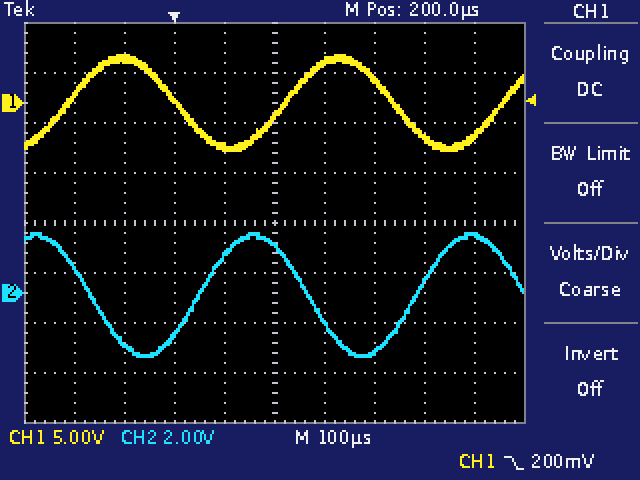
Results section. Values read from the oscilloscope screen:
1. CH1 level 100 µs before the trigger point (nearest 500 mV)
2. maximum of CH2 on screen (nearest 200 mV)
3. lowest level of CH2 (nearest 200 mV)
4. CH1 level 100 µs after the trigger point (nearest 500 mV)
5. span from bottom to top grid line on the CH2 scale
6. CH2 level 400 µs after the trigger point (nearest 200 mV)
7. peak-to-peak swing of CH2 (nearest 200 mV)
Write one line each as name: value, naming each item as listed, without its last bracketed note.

CH1 level 100 µs before the trigger point: 4.5 V
maximum of CH2 on screen: 2.4 V
lowest level of CH2: -2.6 V
CH1 level 100 µs after the trigger point: -4.5 V
span from bottom to top grid line on the CH2 scale: 16 V
CH2 level 400 µs after the trigger point: -2.4 V
peak-to-peak swing of CH2: 5.0 V
